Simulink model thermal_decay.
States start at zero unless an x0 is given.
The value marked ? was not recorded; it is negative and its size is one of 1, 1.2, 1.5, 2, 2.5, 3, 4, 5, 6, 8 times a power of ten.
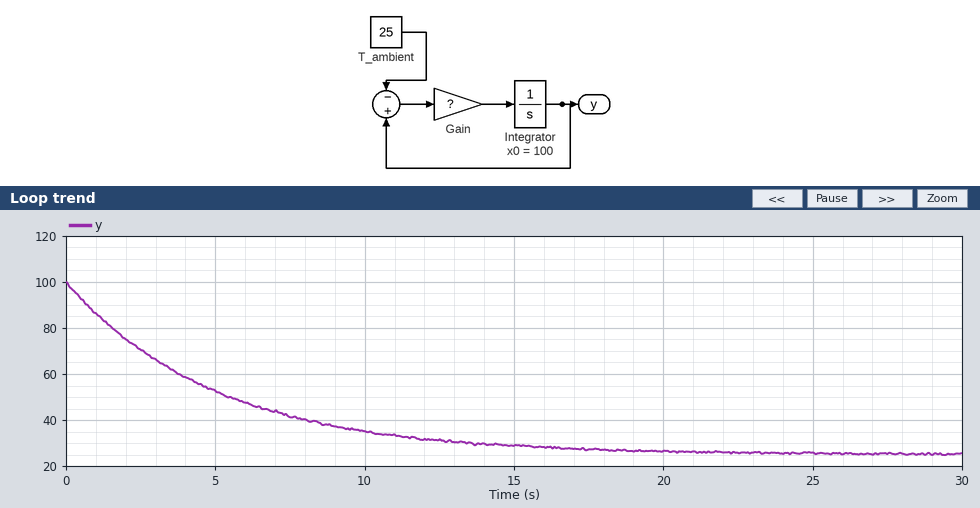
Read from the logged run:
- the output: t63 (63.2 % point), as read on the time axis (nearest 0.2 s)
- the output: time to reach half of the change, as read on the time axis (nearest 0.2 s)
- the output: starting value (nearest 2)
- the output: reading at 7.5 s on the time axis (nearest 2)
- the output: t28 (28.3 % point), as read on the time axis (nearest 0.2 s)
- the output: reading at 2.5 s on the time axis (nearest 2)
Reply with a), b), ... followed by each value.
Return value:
a) 5.0 s
b) 3.4 s
c) 100
d) 42
e) 1.6 s
f) 70
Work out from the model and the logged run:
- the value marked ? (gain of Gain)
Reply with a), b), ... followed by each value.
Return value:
a) -0.2
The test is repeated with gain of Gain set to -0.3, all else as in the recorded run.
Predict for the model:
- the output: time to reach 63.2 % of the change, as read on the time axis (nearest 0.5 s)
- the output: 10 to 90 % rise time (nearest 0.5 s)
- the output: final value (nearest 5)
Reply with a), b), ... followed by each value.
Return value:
a) 3.5 s
b) 7.5 s
c) 25
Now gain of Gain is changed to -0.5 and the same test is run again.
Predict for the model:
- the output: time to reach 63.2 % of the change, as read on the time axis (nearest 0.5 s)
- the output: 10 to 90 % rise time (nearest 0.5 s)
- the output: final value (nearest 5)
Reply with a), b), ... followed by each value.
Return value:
a) 2.0 s
b) 4.5 s
c) 25
